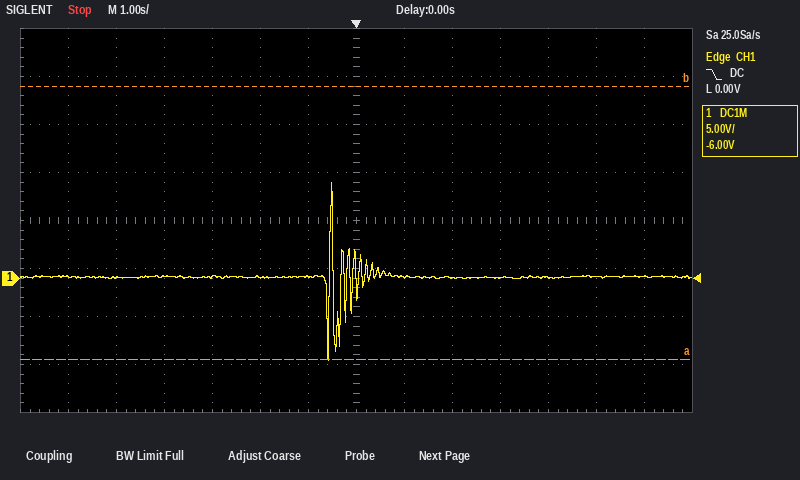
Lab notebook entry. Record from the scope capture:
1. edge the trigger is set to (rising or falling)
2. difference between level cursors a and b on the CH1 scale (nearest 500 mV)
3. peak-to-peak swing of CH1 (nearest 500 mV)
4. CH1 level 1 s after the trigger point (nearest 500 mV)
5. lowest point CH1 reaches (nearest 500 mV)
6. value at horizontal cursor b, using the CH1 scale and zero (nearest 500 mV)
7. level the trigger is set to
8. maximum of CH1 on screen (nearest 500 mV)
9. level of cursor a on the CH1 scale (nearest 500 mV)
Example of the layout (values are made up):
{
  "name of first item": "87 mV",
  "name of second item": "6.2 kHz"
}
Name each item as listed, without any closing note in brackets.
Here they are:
{
  "edge the trigger is set to": "falling",
  "difference between level cursors a and b on the CH1 scale": "28.5 V",
  "peak-to-peak swing of CH1": "18.5 V",
  "CH1 level 1 s after the trigger point": "0.0 V",
  "lowest point CH1 reaches": "-8.5 V",
  "value at horizontal cursor b, using the CH1 scale and zero": "20.0 V",
  "level the trigger is set to": "0.00 V",
  "maximum of CH1 on screen": "10.0 V",
  "level of cursor a on the CH1 scale": "-8.5 V"
}
